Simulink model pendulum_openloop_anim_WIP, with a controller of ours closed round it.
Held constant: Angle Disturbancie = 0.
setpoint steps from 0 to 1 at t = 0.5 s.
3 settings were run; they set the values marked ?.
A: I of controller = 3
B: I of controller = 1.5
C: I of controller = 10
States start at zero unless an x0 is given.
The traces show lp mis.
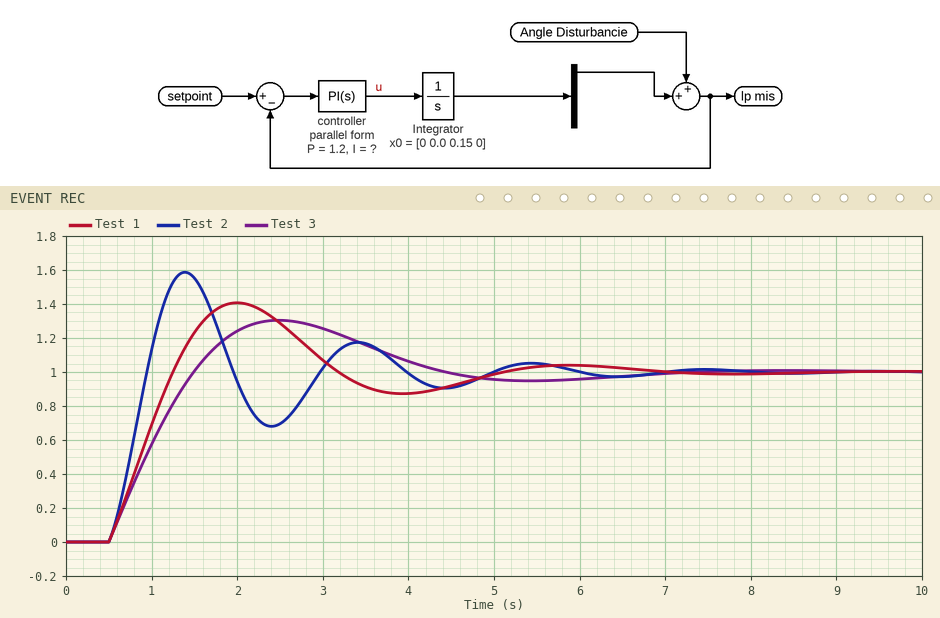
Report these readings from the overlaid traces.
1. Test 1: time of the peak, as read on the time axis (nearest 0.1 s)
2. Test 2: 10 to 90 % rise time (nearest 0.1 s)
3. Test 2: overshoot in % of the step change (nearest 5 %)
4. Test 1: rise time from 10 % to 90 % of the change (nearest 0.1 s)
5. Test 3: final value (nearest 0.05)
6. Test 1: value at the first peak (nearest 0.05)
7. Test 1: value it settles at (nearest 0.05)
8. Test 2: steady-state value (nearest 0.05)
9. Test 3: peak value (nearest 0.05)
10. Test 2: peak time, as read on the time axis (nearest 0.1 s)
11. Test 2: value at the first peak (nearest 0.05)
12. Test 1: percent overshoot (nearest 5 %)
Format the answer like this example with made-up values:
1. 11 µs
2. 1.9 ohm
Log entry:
1. 2.0 s
2. 0.3 s
3. 60 %
4. 0.6 s
5. 1.00
6. 1.40
7. 1.00
8. 1.00
9. 1.30
10. 1.4 s
11. 1.60
12. 40 %
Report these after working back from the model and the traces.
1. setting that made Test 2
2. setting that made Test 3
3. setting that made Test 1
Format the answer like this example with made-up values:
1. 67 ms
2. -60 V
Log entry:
1. C
2. B
3. A
